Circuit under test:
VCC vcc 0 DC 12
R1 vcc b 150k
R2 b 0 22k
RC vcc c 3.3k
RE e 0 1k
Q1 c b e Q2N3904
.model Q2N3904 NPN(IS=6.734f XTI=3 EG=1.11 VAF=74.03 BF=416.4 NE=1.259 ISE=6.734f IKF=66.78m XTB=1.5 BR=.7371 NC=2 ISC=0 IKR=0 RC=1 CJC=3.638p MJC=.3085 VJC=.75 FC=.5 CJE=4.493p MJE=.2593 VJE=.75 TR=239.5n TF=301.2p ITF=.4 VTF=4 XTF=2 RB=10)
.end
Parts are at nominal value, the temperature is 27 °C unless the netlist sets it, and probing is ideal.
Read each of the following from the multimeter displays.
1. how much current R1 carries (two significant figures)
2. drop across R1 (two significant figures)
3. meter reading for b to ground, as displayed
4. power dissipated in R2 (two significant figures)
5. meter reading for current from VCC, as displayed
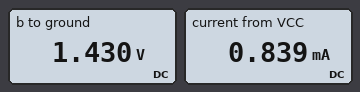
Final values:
70 µA
11 V
1.430 V
93 µW
0.839 mA
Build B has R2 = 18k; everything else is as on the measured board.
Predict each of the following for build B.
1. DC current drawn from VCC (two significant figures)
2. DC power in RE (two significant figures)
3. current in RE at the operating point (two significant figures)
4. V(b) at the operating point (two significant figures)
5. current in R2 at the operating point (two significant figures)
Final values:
640 µA
330 µW
570 µA
1.2 V
68 µA
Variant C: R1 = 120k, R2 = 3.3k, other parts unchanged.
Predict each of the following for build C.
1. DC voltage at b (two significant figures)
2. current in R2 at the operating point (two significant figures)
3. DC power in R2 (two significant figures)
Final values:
320 mV
97 µA
31 µW
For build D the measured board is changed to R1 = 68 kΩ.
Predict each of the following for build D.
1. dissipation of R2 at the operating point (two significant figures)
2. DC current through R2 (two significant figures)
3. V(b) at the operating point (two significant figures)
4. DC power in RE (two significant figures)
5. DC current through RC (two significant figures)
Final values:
330 µW
120 µA
2.7 V
4.1 mW
2.0 mA
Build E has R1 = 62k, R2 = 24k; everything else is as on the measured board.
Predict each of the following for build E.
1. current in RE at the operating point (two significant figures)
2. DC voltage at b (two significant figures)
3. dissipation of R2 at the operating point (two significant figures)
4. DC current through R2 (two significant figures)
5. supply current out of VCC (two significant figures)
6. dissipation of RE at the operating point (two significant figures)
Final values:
2.4 mA
3.1 V
390 µW
130 µA
2.5 mA
5.7 mW
